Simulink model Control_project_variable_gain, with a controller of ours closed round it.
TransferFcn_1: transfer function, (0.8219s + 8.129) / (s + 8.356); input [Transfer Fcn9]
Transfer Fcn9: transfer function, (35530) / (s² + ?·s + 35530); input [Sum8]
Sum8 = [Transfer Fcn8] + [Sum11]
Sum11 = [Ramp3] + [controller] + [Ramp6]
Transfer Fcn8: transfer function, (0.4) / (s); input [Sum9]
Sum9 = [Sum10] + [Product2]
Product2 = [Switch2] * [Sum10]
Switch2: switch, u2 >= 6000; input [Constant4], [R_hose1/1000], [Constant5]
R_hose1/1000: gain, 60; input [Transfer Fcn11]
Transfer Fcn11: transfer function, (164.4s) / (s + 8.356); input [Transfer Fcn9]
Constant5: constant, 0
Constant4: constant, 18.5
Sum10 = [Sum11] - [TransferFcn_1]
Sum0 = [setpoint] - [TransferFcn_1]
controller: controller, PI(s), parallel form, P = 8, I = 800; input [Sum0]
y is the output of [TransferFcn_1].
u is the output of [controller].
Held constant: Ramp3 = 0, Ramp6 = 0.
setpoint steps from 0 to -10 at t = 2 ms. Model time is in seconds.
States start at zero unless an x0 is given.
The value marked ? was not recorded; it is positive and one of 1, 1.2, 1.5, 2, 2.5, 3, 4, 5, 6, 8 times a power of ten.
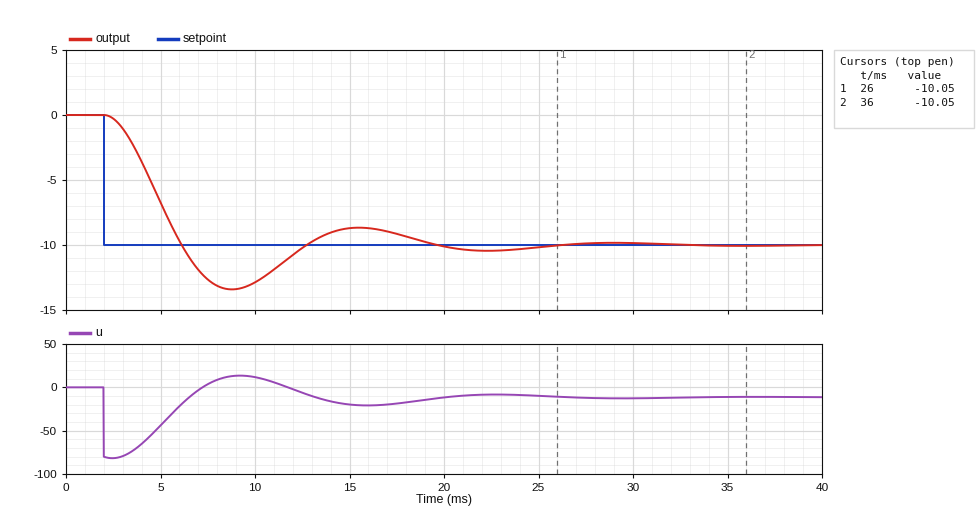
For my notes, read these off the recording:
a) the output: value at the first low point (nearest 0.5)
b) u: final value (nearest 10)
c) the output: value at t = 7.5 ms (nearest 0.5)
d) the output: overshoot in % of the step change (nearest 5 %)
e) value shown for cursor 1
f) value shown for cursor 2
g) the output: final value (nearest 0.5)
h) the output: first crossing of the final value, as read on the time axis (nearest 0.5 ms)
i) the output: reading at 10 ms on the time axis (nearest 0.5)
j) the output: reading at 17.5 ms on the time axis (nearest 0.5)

-13.5
-10
-12.5
35 %
-10.05
-10.05
-10.0
6.0 ms
-13.0
-9.0
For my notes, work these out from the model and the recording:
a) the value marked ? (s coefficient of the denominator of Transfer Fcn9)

400
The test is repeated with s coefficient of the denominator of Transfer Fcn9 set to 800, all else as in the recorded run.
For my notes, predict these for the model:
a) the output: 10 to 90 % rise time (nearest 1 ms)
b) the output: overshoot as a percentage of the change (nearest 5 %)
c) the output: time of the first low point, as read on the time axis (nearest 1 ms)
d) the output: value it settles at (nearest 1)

4 ms
15 %
12 ms
-10
